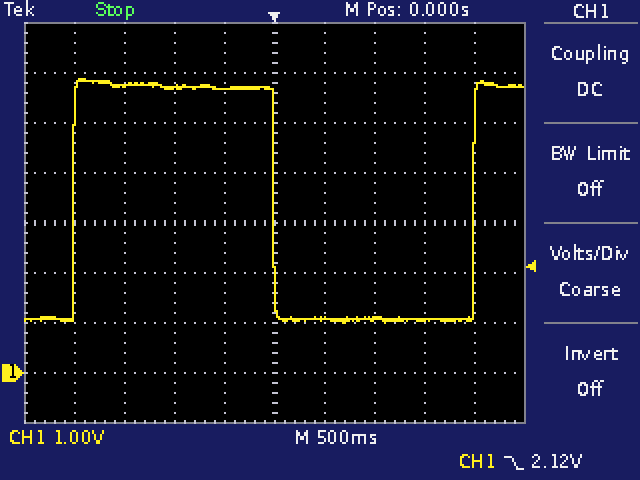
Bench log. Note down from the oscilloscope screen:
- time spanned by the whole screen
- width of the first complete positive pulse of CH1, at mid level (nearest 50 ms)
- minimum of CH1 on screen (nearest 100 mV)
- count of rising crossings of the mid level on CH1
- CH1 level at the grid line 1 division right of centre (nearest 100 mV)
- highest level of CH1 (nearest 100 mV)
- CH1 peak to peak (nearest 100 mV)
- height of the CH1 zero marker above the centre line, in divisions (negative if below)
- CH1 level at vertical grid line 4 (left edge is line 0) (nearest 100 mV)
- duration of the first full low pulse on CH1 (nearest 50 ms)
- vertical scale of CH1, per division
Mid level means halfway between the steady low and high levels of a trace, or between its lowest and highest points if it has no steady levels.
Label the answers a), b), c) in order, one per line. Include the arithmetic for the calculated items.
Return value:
a) 5 s
b) 2.00 s
c) 1.0 V
d) 2
e) 1.1 V
f) 5.9 V
g) 5.9 V − (1.0 V) = 4.9 V
h) -3.0 div
i) 5.7 V
j) 2.00 s
k) 1 V
